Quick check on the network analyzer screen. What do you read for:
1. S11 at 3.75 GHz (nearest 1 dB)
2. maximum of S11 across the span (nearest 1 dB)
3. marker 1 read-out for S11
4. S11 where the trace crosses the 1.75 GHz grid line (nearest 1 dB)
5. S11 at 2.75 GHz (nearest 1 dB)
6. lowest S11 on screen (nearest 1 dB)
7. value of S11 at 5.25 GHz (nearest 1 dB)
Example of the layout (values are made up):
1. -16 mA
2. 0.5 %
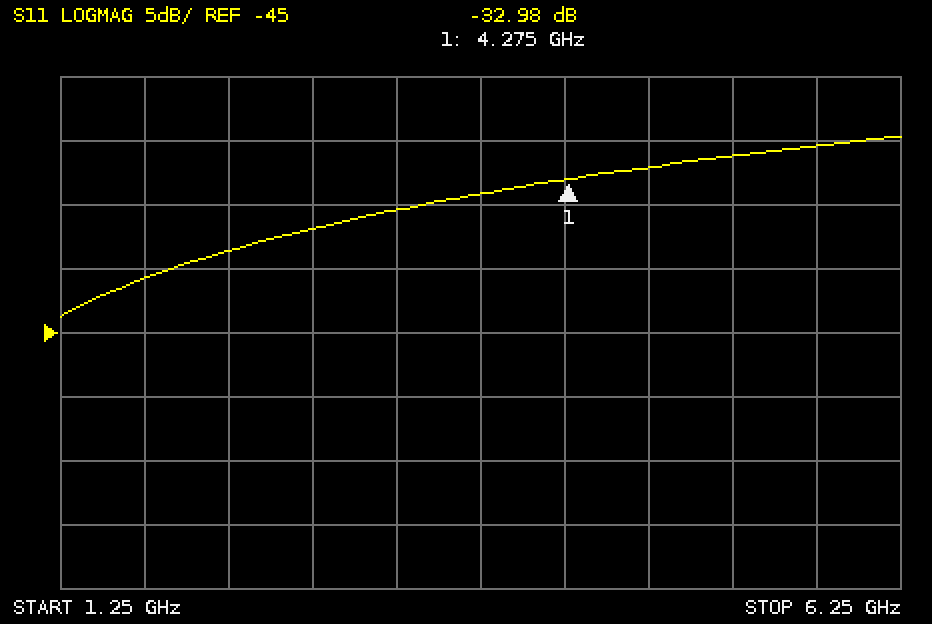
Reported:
1. -34 dB
2. -30 dB
3. -32.98 dB
4. -41 dB
5. -37 dB
6. -44 dB
7. -31 dB
